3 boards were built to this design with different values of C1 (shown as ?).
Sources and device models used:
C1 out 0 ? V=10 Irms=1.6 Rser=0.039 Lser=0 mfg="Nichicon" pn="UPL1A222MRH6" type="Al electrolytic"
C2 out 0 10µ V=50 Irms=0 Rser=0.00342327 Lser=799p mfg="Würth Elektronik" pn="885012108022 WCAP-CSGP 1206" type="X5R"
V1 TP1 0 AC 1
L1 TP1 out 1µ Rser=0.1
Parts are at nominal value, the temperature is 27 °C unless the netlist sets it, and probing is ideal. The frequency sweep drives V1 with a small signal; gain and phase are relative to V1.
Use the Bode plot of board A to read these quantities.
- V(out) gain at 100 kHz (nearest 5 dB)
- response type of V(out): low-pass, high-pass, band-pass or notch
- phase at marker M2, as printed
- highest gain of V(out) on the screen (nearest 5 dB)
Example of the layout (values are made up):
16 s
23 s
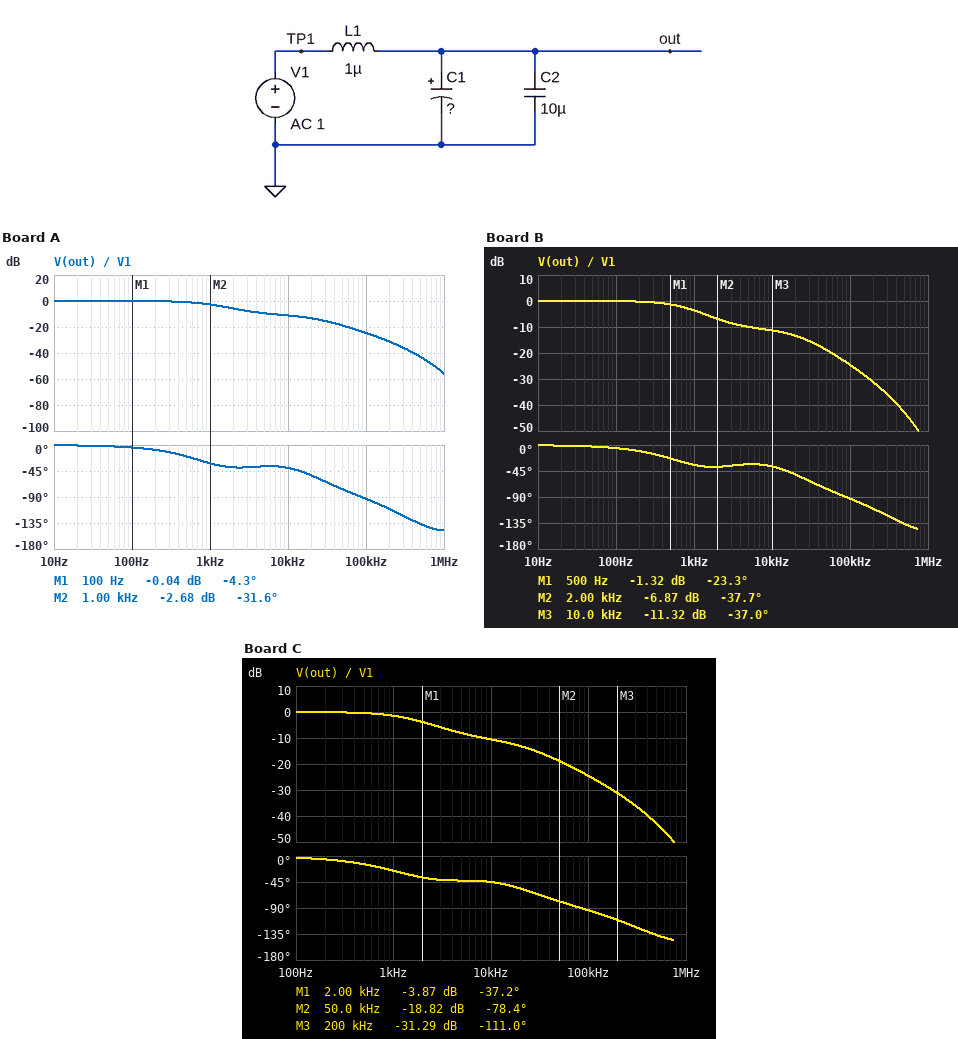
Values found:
-25 dB
low-pass
-31.6 deg
0 dB
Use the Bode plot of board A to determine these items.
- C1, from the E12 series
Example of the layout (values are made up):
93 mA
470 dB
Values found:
1.2 mF
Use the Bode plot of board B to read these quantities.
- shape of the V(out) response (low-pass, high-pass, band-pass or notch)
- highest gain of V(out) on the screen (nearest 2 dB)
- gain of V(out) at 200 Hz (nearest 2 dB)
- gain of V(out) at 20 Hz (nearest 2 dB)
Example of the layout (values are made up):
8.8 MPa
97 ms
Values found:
low-pass
0 dB
0 dB
0 dB
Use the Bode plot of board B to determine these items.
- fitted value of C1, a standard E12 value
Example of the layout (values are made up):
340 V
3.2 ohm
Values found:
1.5 mF
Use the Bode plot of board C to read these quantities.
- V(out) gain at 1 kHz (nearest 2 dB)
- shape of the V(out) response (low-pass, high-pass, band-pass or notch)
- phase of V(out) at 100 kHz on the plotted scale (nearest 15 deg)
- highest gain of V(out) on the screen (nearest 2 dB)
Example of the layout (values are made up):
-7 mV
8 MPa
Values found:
-2 dB
low-pass
-90 deg
0 dB
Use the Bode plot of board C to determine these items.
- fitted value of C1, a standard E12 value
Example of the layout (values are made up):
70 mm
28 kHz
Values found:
820 µF
